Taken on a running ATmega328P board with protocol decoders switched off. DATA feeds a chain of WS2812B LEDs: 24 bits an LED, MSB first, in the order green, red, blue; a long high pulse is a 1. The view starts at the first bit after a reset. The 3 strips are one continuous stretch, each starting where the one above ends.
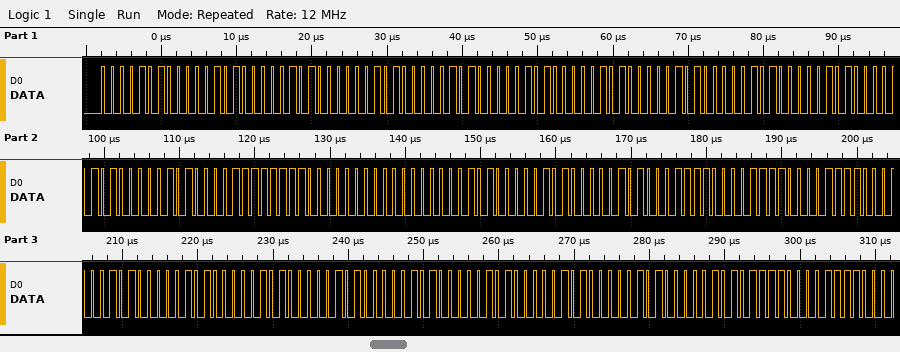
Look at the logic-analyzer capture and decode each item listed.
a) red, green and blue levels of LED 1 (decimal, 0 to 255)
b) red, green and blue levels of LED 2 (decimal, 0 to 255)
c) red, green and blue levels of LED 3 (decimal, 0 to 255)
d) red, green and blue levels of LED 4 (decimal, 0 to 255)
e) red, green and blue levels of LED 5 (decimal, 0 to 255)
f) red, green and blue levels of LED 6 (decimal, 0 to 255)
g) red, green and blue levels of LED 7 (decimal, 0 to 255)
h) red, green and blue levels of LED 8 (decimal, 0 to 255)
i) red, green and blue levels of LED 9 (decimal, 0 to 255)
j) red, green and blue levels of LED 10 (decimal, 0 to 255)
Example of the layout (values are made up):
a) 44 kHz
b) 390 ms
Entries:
a) 10, 10, 10
b) 5, 5, 5
c) 5, 5, 5
d) 5, 5, 5
e) 240, 15, 0
f) 5, 5, 5
g) 30, 30, 30
h) 5, 5, 5
i) 5, 5, 5
j) 5, 5, 5
